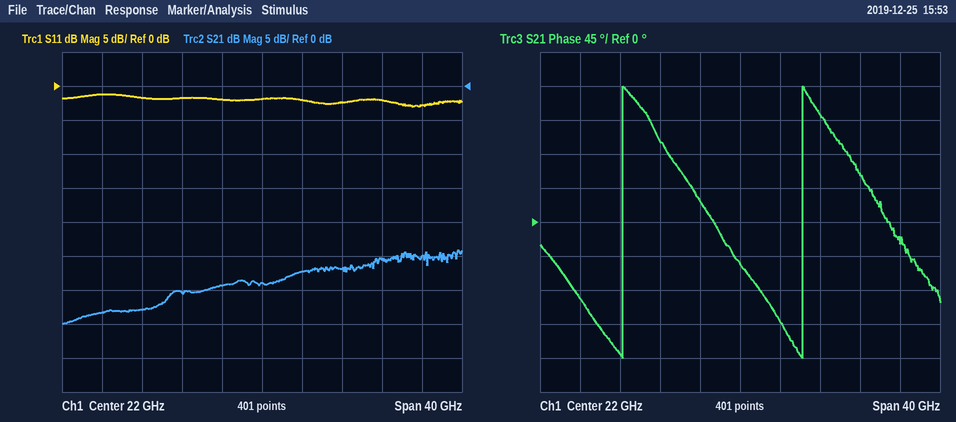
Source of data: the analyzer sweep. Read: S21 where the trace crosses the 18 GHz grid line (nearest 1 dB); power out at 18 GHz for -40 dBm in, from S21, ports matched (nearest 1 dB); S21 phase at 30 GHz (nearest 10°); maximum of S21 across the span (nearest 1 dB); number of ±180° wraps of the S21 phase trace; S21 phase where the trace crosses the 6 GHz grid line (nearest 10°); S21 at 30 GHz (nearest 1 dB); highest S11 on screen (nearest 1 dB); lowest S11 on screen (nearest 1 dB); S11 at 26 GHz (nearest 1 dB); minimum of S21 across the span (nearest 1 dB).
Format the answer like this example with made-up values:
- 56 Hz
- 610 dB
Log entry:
- -29 dB
- -69 dBm
- 140°
- -24 dB
- 2
- -100°
- -27 dB
- -1 dB
- -3 dB
- -2 dB
- -35 dB
